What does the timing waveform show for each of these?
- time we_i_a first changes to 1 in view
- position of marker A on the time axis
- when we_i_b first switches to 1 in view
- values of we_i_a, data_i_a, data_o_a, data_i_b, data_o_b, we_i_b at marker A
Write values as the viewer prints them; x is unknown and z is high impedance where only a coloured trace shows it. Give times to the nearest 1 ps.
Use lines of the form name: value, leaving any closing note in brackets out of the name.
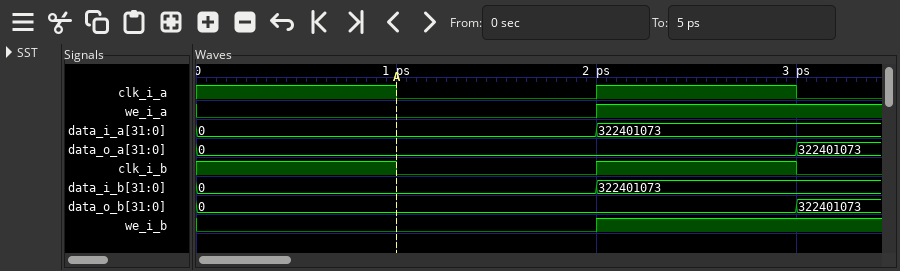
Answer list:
time we_i_a first changes to 1 in view: 2 ps
position of marker A on the time axis: 1 ps
when we_i_b first switches to 1 in view: 2 ps
values of we_i_a, data_i_a, data_o_a, data_i_b, data_o_b, we_i_b at marker A: we_i_a=0, data_i_a=0, data_o_a=0, data_i_b=0, data_o_b=0, we_i_b=0
